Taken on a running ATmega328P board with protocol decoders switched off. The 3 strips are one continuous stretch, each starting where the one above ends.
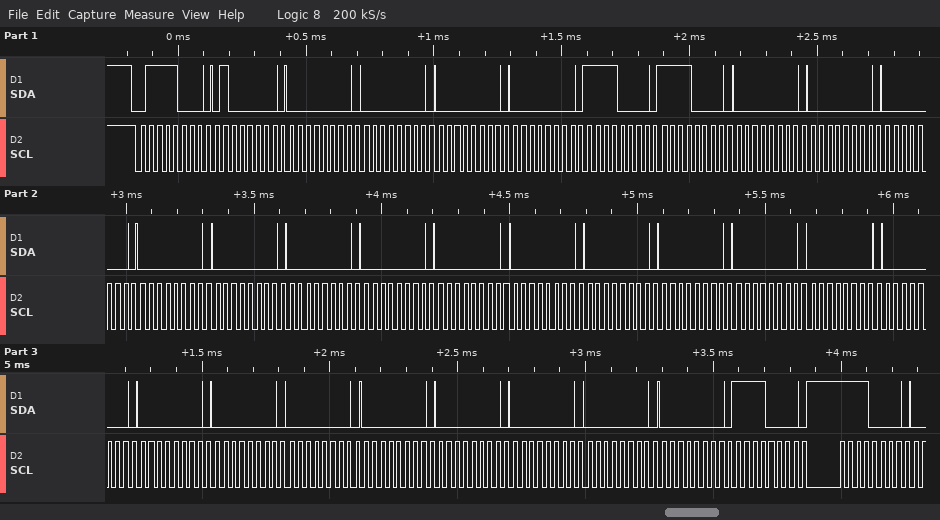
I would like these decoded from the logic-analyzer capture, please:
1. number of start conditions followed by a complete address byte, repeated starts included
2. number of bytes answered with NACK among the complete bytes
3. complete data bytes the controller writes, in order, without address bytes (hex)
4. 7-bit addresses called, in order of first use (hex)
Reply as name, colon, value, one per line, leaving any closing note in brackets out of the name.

number of start conditions followed by a complete address byte, repeated starts included: 1
number of bytes answered with NACK among the complete bytes: 0
complete data bytes the controller writes, in order, without address bytes: 40 00 00 00 00 F0 F0 00 00 00 00 00 00 00 00 00 00 00 00 00 00 00 00 00 00 00 00 00 00 F0 F0
7-bit addresses called, in order of first use: 0x3C
